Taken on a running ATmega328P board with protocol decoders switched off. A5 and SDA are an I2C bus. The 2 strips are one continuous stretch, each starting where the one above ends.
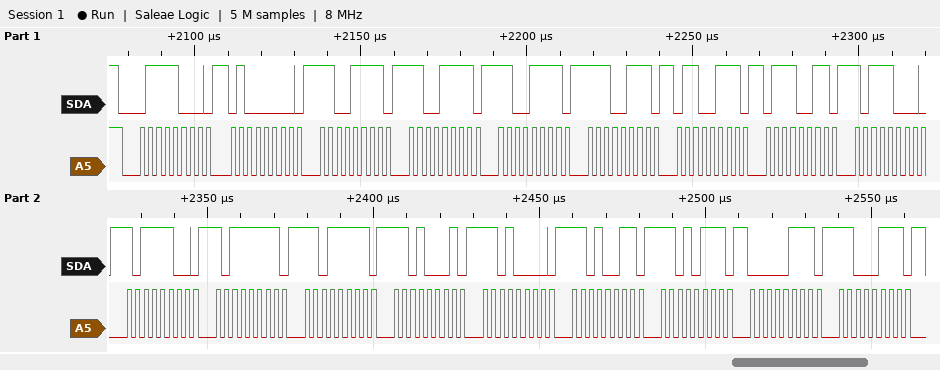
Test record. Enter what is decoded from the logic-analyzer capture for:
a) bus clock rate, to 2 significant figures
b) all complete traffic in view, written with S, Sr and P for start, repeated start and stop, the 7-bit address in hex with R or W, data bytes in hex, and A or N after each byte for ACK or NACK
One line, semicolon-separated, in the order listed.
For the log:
400 kHz; S 3CW A 40 A CF A CF A CF A E7 A 67 A 73 A B8 A BC A BF A DF A D1 A D0 A D3 A D7 A 07 A C7 A
